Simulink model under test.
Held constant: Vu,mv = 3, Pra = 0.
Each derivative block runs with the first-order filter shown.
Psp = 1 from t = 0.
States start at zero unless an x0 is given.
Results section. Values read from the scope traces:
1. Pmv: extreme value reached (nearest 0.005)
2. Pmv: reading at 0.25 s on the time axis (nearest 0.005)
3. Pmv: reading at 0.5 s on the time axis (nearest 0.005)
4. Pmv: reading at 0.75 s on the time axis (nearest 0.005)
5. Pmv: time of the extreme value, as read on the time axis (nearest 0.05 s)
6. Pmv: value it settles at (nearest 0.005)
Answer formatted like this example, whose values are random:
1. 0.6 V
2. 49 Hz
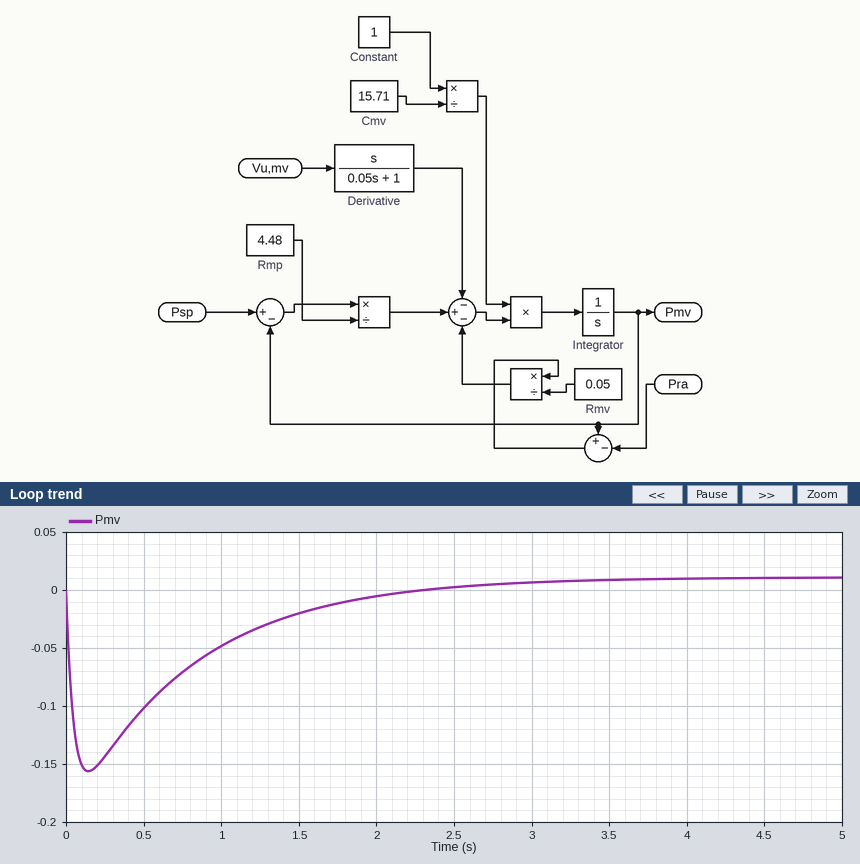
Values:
1. -0.155
2. -0.145
3. -0.100
4. -0.070
5. 0.15 s
6. 0.010
